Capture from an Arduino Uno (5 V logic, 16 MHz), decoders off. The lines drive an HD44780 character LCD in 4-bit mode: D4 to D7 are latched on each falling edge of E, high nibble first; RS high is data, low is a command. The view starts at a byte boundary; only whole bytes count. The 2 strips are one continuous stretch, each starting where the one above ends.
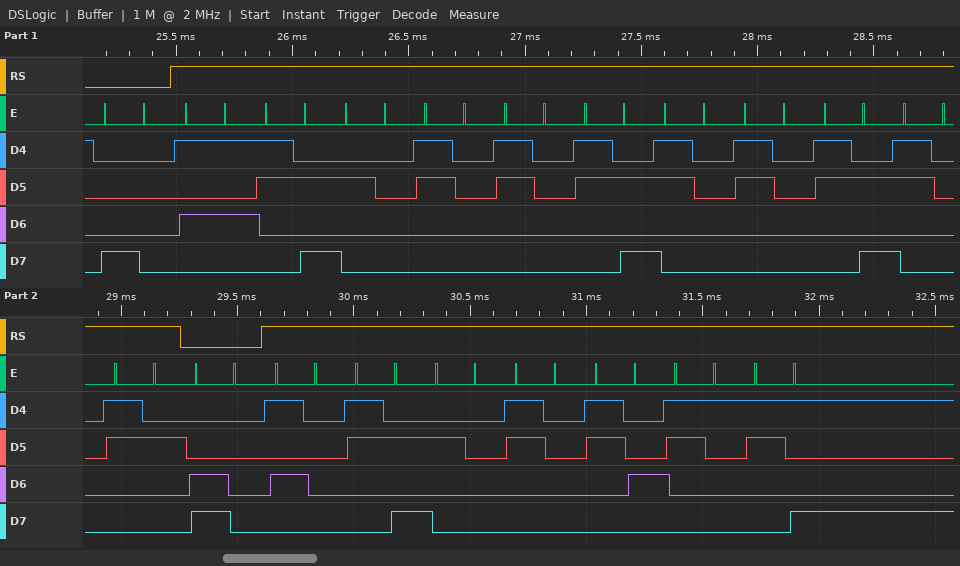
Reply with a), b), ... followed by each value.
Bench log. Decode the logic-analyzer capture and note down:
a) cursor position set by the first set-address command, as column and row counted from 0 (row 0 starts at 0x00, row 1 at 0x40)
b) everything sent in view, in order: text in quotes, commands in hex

a) column 0, row 0
b) 0x80 "U: 00:00:02" 0xC0 "P: 0419"
